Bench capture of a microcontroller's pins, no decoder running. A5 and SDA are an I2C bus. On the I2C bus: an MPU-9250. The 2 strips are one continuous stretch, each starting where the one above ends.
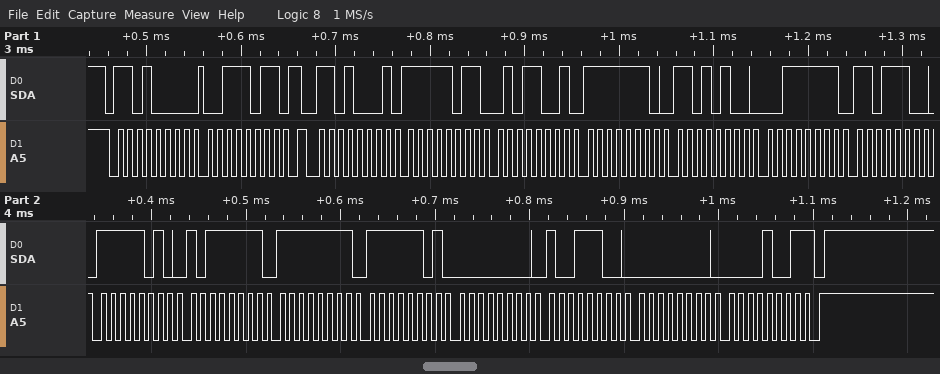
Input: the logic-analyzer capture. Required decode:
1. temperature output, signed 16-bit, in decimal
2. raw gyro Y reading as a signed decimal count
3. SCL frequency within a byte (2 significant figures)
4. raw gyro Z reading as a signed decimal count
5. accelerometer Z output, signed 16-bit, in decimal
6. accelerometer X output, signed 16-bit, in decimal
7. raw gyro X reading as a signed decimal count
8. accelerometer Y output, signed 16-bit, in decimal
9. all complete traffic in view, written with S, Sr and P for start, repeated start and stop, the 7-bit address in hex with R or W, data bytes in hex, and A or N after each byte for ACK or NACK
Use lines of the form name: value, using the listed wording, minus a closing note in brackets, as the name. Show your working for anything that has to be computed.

temperature output, signed 16-bit, in decimal: 0xFABF = -1345
raw gyro Y reading as a signed decimal count: 0x009C = 156
SCL frequency within a byte: 100 kHz
raw gyro Z reading as a signed decimal count: 0x0009 = 9
accelerometer Z output, signed 16-bit, in decimal: 0x3FDC = 16348
accelerometer X output, signed 16-bit, in decimal: 0xFB59 = -1191
raw gyro X reading as a signed decimal count: 0xFFFD = -3
accelerometer Y output, signed 16-bit, in decimal: 0xFED4 = -300
all complete traffic in view, written with S, Sr and P for start, repeated start and stop, the 7-bit address in hex with R or W, data bytes in hex, and A or N after each byte for ACK or NACK: S 68W A 3B A Sr 68R A FB A 59 A FE A D4 A 3F A DC A FA A BF A FF A FD A 00 A 9C A 00 A 09 N P
